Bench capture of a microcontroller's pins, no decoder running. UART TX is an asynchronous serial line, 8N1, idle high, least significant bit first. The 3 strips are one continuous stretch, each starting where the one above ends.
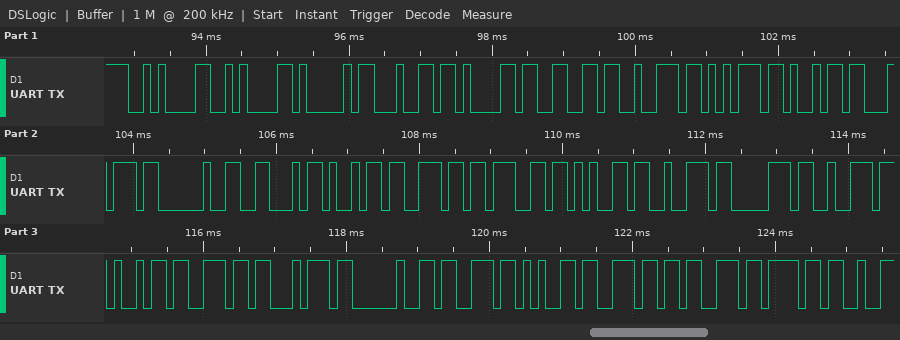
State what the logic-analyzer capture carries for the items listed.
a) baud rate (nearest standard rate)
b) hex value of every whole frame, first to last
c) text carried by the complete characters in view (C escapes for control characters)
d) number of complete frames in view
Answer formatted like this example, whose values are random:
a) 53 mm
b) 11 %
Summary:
a) 9600 baud
b) 0A 0A 41 64 61 66 72 75 69 74 20 46 69 6E 67 65 72 70 72 69 6E 74 20 73 65 6E 73 6F
c) "\n\nAdafruit Fingerprint senso"
d) 28
